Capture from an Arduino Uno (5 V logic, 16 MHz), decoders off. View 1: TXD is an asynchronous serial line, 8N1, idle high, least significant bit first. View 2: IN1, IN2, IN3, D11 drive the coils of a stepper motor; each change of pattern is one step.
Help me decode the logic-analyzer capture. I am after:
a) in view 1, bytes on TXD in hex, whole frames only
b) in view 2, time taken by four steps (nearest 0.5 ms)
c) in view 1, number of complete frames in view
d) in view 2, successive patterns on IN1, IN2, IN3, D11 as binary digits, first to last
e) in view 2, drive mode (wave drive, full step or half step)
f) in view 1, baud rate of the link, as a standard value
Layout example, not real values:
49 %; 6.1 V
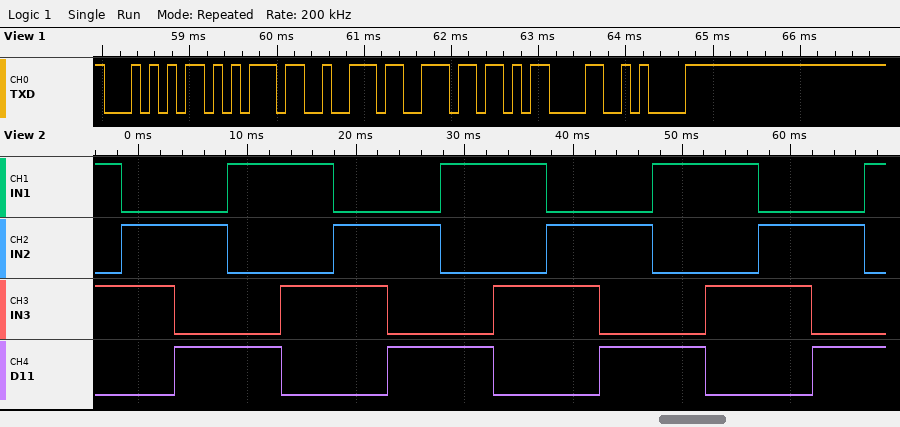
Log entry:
54 75 72 6E 0D 0A; 19.5 ms; 6; 1010 0110 0101 1001 1010 0110 0101 1001 1010 0110 0101 1001 1010 0110 0101 1001; full step; 9600 baud
